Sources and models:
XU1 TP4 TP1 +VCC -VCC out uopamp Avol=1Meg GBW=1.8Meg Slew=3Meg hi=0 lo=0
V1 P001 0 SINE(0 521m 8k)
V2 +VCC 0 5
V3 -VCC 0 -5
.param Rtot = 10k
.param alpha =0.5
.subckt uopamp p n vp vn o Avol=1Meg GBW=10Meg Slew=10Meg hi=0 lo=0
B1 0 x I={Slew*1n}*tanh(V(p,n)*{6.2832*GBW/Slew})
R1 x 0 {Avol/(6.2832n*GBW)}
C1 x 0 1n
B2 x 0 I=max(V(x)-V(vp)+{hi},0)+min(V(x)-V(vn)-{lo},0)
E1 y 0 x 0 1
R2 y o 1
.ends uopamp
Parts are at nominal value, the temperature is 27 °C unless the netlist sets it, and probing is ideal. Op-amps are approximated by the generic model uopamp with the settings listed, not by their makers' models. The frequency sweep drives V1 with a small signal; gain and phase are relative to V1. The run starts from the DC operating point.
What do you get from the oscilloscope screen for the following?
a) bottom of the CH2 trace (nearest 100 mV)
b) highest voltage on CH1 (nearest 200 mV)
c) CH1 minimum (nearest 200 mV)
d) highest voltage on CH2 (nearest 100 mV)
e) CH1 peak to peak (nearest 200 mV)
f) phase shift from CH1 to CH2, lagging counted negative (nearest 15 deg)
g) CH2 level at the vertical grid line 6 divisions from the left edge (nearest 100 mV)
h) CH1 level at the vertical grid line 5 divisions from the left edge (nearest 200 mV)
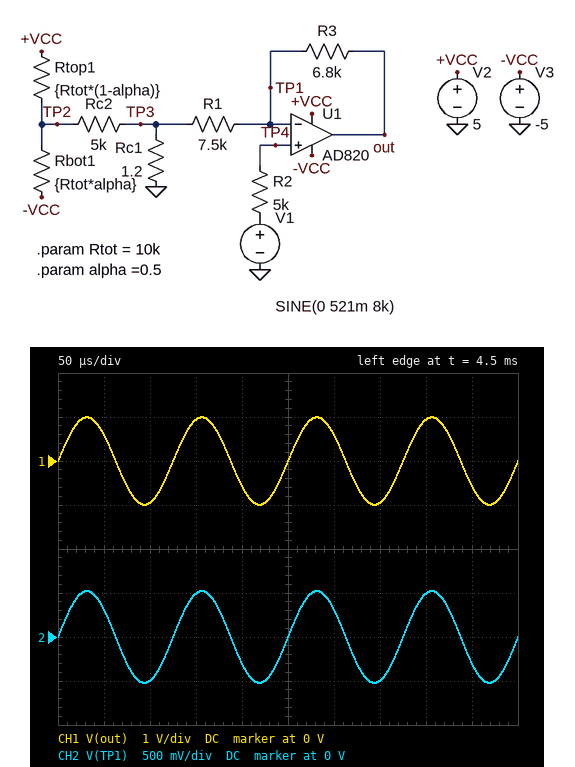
-500 mV
1.0 V
-1.0 V
500 mV
2.0 V
0 deg
300 mV
0 V
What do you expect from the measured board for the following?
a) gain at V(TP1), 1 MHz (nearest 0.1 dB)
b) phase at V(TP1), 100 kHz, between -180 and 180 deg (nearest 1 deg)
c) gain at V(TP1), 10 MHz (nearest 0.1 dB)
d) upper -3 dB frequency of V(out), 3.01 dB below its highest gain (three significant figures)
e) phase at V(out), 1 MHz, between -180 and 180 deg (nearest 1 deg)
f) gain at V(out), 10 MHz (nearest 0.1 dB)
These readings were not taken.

-3.3 dB
-6 deg
-20.5 dB
944 kHz
-47 deg
-14.9 dB
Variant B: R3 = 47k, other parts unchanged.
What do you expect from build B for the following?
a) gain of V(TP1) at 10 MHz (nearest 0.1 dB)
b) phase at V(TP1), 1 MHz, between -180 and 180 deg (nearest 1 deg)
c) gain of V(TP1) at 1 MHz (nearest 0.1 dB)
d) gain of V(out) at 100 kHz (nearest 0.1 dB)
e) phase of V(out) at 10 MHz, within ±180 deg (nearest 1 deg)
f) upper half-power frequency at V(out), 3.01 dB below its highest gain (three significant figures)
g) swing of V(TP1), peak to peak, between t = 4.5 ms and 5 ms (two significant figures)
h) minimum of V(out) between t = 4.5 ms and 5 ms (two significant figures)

-32.1 dB
-76 deg
-12.4 dB
16.6 dB
-89 deg
248 kHz
1.0 V
-3.8 V
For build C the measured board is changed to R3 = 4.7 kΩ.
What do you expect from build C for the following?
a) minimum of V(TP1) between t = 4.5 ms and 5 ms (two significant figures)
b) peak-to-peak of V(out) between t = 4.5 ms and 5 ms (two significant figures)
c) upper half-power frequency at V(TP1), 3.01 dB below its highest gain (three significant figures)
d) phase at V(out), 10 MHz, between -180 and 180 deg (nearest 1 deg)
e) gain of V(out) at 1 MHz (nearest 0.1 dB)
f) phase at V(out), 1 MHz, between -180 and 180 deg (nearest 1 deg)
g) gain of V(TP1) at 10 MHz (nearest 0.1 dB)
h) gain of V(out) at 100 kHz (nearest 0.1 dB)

-520 mV
1.7 V
1.11 MHz
-84 deg
1.6 dB
-42 deg
-19.2 dB
4.2 dB
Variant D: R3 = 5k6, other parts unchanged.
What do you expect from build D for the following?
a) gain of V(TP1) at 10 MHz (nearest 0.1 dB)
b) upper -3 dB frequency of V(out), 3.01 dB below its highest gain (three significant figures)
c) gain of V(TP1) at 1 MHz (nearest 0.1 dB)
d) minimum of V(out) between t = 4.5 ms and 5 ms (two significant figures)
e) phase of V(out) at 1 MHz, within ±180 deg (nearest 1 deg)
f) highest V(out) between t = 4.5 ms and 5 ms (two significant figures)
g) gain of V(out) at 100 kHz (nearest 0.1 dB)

-19.8 dB
1.03 MHz
-2.9 dB
-910 mV
-44 deg
910 mV
4.8 dB
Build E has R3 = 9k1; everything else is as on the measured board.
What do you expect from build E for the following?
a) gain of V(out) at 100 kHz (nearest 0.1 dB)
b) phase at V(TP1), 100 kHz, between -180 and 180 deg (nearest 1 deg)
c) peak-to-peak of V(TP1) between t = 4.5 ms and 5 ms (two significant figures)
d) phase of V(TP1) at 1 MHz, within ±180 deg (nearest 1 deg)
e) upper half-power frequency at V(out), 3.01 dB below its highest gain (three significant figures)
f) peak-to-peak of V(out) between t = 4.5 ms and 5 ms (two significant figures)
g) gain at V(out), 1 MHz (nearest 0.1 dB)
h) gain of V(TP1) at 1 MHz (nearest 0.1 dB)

6.8 dB
-7 deg
1.0 V
-51 deg
813 kHz
2.3 V
2.9 dB
-4.0 dB
